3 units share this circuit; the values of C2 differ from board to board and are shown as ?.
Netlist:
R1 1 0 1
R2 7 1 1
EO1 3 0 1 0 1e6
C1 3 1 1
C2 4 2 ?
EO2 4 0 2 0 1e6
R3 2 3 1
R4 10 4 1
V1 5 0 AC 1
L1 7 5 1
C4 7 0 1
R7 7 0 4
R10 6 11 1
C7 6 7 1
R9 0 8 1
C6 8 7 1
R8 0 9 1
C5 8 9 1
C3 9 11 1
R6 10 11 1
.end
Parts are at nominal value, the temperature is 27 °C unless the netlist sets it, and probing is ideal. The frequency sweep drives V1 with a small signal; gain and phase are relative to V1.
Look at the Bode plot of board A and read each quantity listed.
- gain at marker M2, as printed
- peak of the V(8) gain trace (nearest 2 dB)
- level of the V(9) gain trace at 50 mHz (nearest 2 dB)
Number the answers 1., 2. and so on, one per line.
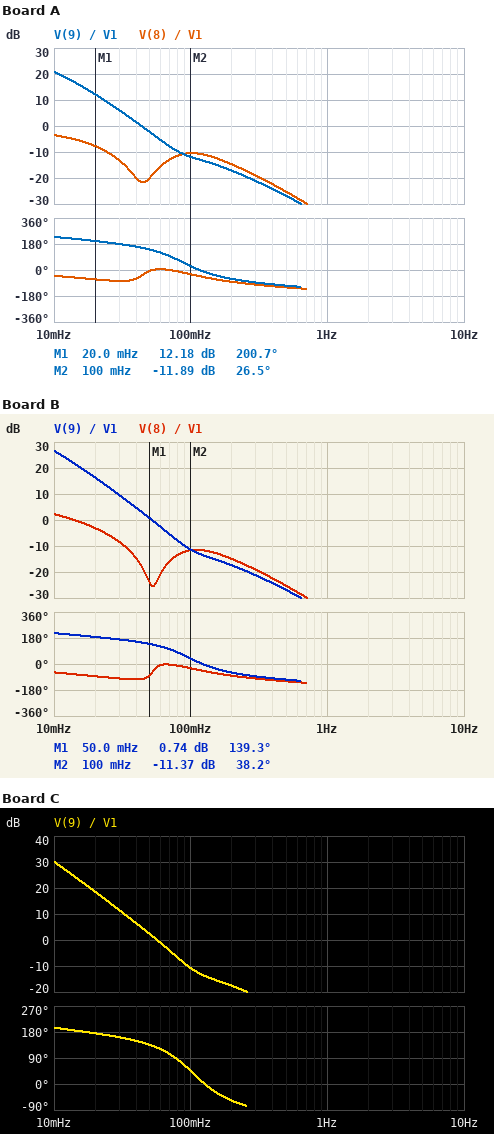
1. -11.89 dB
2. -4 dB
3. -2 dB
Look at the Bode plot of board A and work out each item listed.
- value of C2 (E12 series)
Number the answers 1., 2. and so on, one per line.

1. 2.2 F
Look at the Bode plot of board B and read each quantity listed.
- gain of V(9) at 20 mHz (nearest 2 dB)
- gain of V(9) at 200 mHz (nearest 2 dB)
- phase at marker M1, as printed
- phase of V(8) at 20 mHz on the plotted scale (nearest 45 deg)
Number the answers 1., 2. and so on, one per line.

1. 16 dB
2. -18 dB
3. 139.3 deg
4. -90 deg
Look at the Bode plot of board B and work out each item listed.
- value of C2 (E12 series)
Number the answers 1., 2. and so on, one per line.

1. 1.5 F
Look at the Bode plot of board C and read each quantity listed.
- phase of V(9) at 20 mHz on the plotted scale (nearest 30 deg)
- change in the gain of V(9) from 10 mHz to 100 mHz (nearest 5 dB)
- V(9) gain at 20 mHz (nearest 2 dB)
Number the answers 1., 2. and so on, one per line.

1. 180 deg
2. -40 dB
3. 18 dB
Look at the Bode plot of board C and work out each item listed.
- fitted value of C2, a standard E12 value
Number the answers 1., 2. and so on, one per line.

1. 1.2 F
